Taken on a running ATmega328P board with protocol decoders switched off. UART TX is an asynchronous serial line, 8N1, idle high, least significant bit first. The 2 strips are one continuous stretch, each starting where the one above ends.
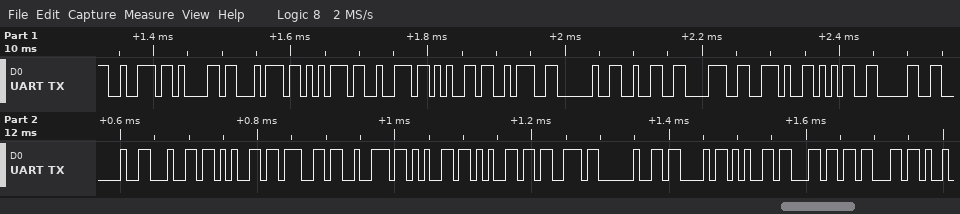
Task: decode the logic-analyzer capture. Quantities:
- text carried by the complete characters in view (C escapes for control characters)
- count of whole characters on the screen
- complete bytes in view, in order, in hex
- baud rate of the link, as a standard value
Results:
"rature: 28.50 degrees Celc"
26
72 61 74 75 72 65 3A 20 32 38 2E 35 30 20 64 65 67 72 65 65 73 20 43 65 6C 63
115200 baud
